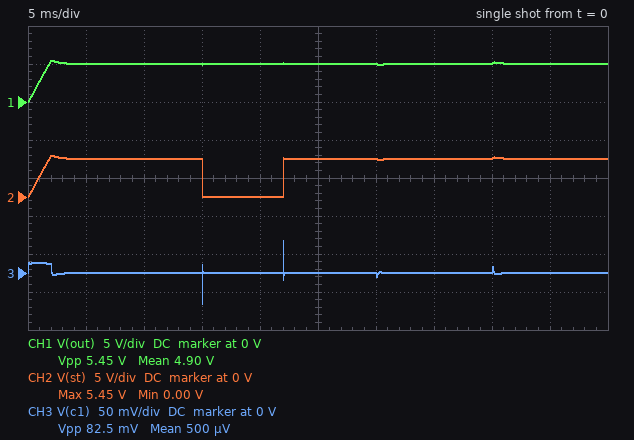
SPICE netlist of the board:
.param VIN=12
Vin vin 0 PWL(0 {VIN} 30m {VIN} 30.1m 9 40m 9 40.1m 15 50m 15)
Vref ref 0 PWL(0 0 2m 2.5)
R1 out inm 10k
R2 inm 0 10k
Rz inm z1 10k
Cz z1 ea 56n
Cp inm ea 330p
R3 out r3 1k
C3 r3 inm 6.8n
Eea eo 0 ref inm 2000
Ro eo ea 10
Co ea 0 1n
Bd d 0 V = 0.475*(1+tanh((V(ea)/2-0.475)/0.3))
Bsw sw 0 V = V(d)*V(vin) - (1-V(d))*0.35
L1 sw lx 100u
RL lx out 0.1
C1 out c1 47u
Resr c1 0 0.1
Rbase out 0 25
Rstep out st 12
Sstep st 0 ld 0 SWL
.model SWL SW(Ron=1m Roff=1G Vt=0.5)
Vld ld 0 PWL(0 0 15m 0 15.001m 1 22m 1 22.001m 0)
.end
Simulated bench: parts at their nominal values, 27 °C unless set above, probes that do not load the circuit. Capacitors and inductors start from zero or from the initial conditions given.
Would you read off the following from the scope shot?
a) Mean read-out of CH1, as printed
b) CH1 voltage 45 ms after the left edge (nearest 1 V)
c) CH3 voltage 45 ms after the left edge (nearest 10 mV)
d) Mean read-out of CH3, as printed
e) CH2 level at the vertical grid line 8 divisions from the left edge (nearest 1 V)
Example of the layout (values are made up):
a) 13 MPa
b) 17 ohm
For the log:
a) 4.90 V
b) 5 V
c) 0 V
d) 500 µV
e) 5 V
